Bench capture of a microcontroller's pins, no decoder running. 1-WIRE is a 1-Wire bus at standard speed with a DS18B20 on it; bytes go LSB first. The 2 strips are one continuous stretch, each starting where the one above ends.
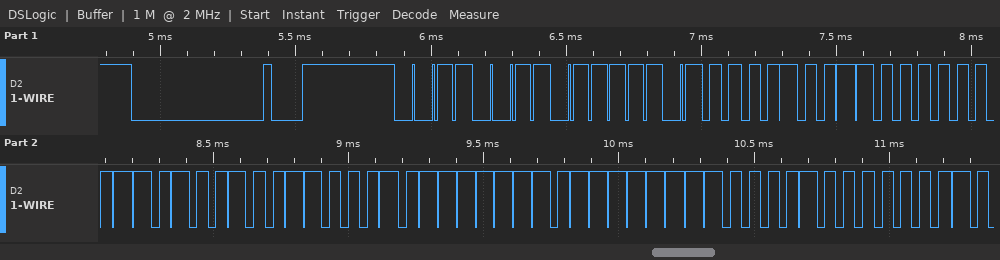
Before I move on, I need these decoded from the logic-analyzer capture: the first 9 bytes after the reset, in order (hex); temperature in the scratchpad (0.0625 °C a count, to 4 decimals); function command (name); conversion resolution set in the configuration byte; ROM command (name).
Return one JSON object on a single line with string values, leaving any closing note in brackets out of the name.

{"the first 9 bytes after the reset, in order": "CC BE 90 01 4B 46 7F FF 10", "temperature in the scratchpad": "25.0000 °C", "function command": "Read Scratchpad", "conversion resolution set in the configuration byte": "12 bits", "ROM command": "Skip ROM"}
